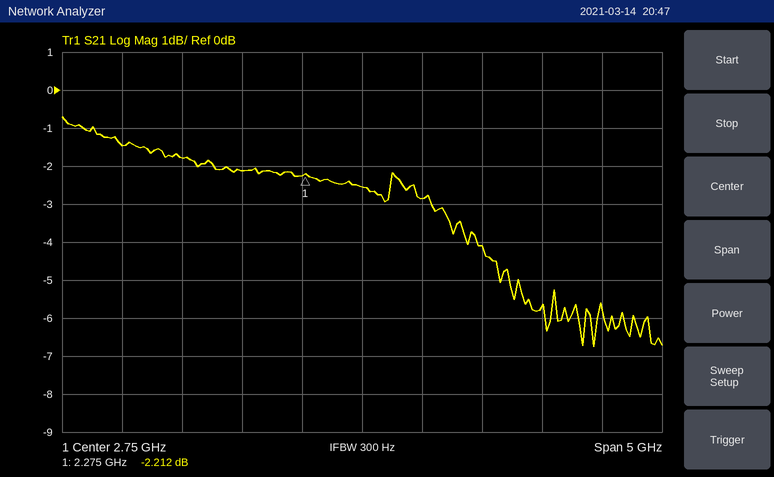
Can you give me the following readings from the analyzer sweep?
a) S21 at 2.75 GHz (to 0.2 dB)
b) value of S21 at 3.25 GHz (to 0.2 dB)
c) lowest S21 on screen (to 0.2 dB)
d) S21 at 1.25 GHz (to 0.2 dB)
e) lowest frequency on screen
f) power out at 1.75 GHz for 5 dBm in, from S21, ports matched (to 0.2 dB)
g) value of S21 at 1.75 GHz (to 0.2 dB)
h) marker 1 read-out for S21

-2.6 dB
-2.8 dB
-6.8 dB
-1.8 dB
250 MHz
2.8 dBm
-2.2 dB
-2.212 dB
